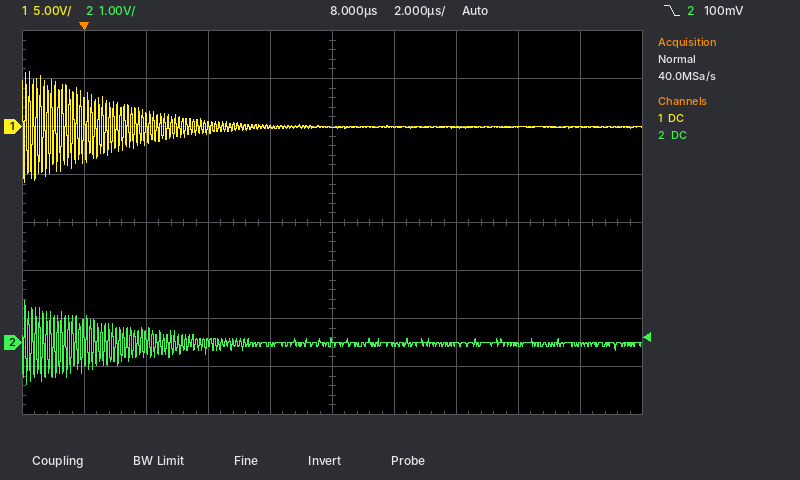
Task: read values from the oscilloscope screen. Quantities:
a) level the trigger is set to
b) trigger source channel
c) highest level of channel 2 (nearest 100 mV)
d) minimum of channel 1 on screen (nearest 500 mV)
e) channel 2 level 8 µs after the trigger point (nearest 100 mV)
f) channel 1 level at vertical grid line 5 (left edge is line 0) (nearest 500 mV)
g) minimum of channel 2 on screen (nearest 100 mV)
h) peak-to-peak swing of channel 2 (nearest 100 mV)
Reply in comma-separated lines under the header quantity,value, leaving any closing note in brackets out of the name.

quantity,value
level the trigger is set to,100 mV
trigger source channel,channel 2
highest level of channel 2,900 mV
minimum of channel 1 on screen,-6.0 V
channel 2 level 8 µs after the trigger point,0.0 V
channel 1 level at vertical grid line 5 (left edge is line 0),0.0 V
minimum of channel 2 on screen,-900 mV
peak-to-peak swing of channel 2,1.8 V
